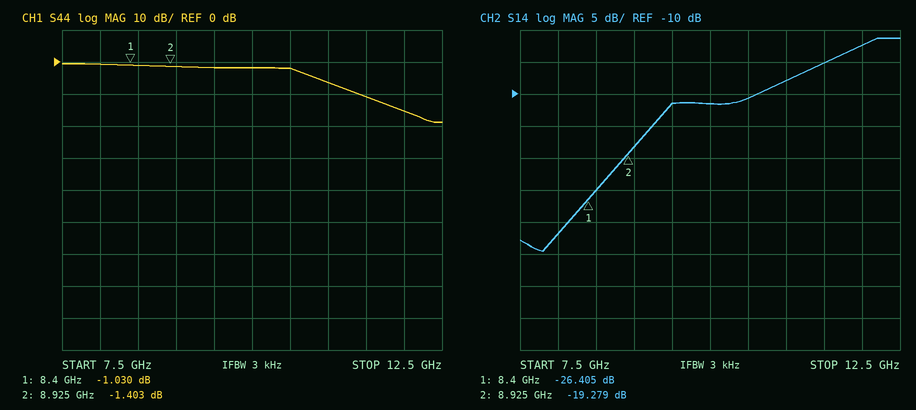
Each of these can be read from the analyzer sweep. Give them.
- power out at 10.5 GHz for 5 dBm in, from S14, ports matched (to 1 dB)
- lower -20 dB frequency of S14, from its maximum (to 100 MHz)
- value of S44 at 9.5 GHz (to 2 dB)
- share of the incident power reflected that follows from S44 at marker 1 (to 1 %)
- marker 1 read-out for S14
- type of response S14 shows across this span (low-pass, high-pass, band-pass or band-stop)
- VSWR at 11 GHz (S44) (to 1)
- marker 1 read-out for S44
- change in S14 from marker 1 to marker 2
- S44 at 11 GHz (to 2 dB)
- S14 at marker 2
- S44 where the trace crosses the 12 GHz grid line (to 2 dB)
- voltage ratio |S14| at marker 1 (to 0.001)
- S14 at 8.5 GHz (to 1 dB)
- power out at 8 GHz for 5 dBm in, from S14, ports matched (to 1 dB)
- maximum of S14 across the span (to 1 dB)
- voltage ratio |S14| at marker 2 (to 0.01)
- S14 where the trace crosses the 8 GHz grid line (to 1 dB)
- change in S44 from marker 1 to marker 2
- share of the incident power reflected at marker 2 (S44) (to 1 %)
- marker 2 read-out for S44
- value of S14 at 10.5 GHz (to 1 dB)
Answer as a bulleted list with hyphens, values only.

- -6 dBm
- 8.8 GHz
- -2 dB
- 79 %
- -26.405 dB
- high-pass
- 3
- -1.030 dB
- 7.126 dB
- -6 dB
- -19.279 dB
- -16 dB
- 0.048
- -25 dB
- -27 dBm
- -1 dB
- 0.11
- -32 dB
- -0.373 dB
- 72 %
- -1.403 dB
- -11 dB
